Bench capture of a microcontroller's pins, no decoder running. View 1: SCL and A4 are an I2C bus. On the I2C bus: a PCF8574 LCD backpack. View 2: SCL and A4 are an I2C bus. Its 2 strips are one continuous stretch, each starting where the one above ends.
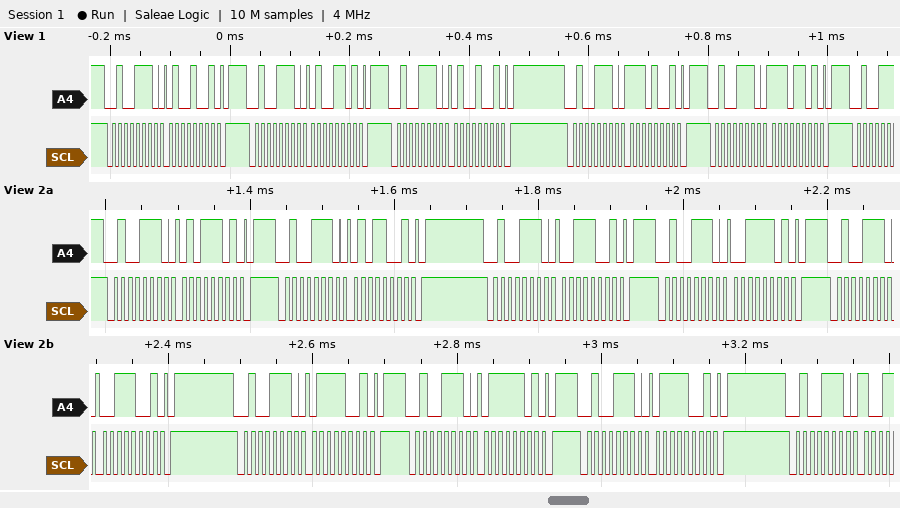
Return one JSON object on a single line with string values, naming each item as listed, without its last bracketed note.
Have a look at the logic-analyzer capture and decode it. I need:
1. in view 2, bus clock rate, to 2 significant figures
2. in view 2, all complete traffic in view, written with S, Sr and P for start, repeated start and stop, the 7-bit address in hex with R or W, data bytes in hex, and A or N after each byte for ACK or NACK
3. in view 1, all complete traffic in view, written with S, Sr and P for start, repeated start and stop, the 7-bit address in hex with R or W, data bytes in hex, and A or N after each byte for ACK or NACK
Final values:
{"in view 2, bus clock rate, to 2 significant figures": "100 kHz", "in view 2, all complete traffic in view, written with S, Sr and P for start, repeated start and stop, the 7-bit address in hex with R or W, data bytes in hex, and A or N after each byte for ACK or NACK": "S 27W A 5D A P S 27W A 59 A P S 27W A 39 A P S 27W A 3D A P S 27W A 39 A P S 27W A 79 A P S 27W A 7D A P S 27W A 79 A P S 27W A", "in view 1, all complete traffic in view, written with S, Sr and P for start, repeated start and stop, the 7-bit address in hex with R or W, data bytes in hex, and A or N after each byte for ACK or NACK": "S 27W A 49 A P S 27W A 4D A P S 27W A 49 A P S 27W A E9 A P S 27W A ED A P"}
